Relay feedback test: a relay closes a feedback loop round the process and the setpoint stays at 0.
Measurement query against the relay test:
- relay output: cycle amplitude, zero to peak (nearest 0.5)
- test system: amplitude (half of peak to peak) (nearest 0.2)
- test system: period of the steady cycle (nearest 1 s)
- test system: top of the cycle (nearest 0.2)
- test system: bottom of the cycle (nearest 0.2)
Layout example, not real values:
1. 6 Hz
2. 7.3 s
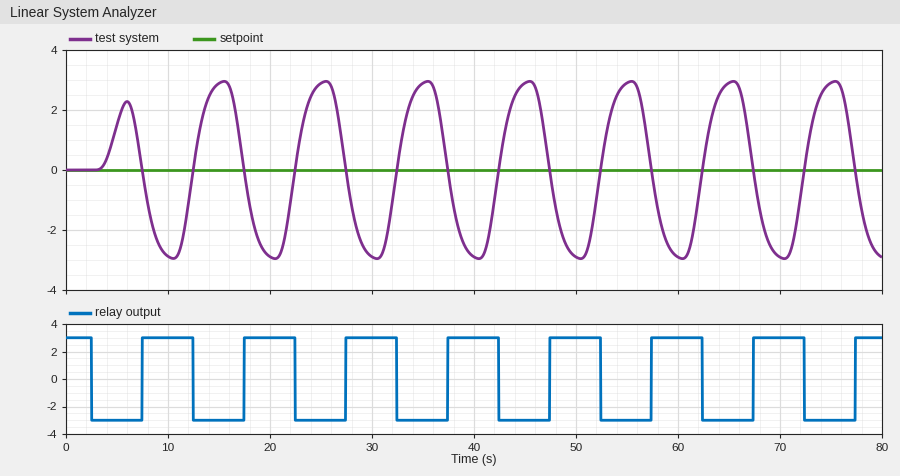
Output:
1. 3.0
2. 3.0
3. 10 s
4. 3.0
5. -3.0
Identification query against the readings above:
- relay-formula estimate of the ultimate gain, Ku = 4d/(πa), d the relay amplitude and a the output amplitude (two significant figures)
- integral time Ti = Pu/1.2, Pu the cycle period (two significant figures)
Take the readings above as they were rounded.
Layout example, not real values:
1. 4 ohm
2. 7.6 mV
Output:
1. 1.3
2. 8.3 s
